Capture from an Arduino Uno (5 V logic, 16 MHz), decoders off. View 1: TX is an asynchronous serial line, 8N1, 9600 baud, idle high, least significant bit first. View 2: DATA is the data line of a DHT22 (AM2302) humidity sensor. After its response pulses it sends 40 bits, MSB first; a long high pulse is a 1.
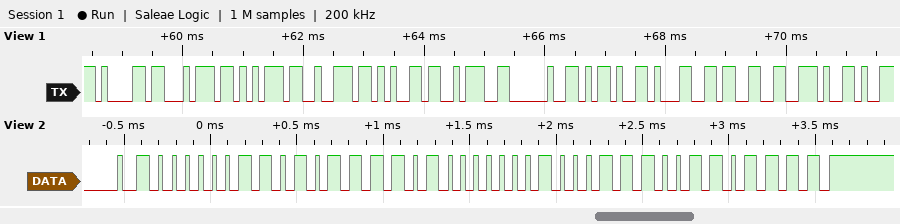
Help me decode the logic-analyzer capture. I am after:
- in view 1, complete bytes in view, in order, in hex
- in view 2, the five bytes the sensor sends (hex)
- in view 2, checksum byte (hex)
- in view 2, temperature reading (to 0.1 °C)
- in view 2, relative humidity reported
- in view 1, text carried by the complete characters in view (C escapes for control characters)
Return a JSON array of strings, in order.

["0x61 0x74 0x75 0x72 0x65 0x3A 0x20 0x2D 0x31 0x33 0x2E", "03 5E 80 8E 6F", "0x6F", "-14.2 °C", "86.2 %", "\"ature: -13.\""]
